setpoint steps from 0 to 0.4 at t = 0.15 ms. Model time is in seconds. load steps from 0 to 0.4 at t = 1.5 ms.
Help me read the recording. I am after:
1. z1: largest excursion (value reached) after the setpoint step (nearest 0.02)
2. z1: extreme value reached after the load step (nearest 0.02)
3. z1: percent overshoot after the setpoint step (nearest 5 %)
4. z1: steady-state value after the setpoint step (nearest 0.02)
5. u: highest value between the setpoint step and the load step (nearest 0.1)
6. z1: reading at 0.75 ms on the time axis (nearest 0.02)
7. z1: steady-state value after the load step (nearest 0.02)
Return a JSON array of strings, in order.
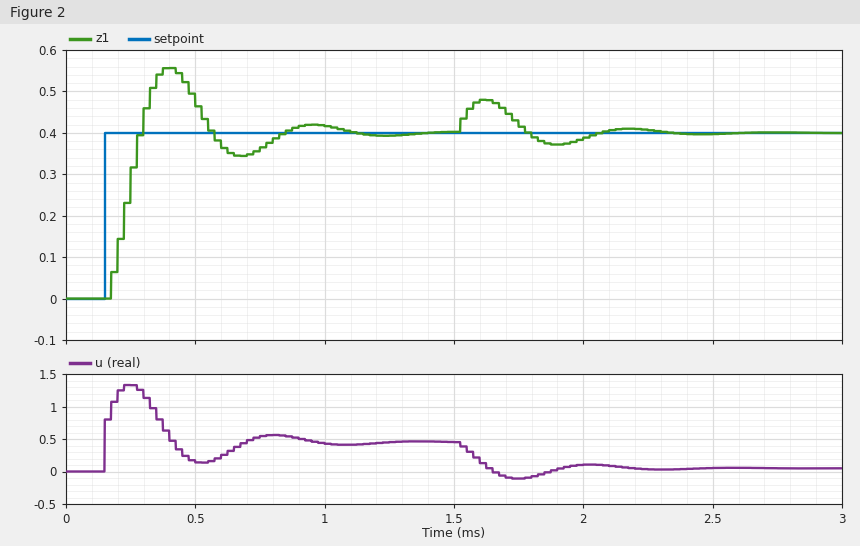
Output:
["0.56", "0.48", "40 %", "0.40", "1.3", "0.36", "0.40"]
